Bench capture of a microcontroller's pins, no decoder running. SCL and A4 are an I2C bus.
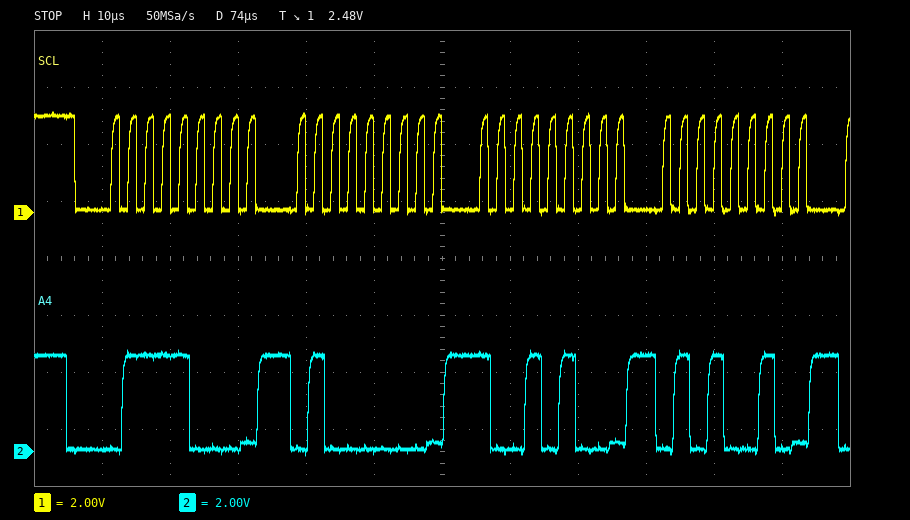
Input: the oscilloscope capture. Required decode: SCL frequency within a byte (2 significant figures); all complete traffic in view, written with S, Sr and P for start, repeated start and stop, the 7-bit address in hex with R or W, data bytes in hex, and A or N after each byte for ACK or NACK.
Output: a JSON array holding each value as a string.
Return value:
["400 kHz", "S 3CW A 40 A 94 A 52 A"]
